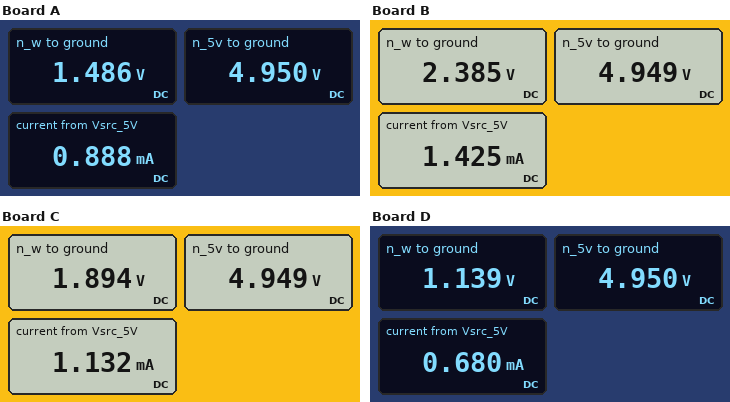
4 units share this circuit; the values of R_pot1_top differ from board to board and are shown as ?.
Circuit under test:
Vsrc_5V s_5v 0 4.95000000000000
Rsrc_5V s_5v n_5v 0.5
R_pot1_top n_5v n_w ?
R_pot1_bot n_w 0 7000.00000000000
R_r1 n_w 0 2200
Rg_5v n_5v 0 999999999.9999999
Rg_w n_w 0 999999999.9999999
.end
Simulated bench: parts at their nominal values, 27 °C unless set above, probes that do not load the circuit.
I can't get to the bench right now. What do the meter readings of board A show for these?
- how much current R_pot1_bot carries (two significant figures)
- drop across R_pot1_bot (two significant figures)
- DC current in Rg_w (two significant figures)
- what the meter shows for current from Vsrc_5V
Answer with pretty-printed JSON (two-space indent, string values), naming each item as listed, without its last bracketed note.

{
  "how much current R_pot1_bot carries": "210 µA",
  "drop across R_pot1_bot": "1.5 V",
  "DC current in Rg_w": "1.5 nA",
  "what the meter shows for current from Vsrc_5V": "0.888 mA"
}
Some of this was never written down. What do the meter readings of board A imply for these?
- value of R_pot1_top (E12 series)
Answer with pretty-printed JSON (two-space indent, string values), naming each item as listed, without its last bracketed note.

{
  "value of R_pot1_top": "3.9 kΩ"
}
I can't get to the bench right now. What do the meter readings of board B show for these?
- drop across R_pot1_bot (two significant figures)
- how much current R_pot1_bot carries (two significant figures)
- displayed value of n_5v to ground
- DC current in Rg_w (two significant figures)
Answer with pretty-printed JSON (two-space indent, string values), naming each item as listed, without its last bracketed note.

{
  "drop across R_pot1_bot": "2.4 V",
  "how much current R_pot1_bot carries": "340 µA",
  "displayed value of n_5v to ground": "4.949 V",
  "DC current in Rg_w": "2.4 nA"
}
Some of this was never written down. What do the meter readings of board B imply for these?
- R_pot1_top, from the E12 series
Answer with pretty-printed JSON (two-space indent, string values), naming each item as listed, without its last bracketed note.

{
  "R_pot1_top, from the E12 series": "1.8 kΩ"
}
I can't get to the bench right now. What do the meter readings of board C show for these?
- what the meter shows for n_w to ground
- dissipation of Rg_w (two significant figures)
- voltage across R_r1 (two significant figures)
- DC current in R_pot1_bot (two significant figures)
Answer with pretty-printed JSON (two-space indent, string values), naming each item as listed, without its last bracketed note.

{
  "what the meter shows for n_w to ground": "1.894 V",
  "dissipation of Rg_w": "3.6 nW",
  "voltage across R_r1": "1.9 V",
  "DC current in R_pot1_bot": "270 µA"
}
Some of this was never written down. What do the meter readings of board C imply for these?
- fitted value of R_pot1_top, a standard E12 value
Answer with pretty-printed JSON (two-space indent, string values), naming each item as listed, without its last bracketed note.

{
  "fitted value of R_pot1_top, a standard E12 value": "2.7 kΩ"
}
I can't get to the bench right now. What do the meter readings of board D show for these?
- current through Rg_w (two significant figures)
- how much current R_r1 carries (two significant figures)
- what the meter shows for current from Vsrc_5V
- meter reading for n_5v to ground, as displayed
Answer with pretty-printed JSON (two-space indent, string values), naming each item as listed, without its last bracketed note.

{
  "current through Rg_w": "1.1 nA",
  "how much current R_r1 carries": "520 µA",
  "what the meter shows for current from Vsrc_5V": "0.680 mA",
  "meter reading for n_5v to ground, as displayed": "4.950 V"
}
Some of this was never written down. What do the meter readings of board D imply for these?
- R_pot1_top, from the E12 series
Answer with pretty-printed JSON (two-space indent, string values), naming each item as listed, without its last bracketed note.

{
  "R_pot1_top, from the E12 series": "5.6 kΩ"
}
